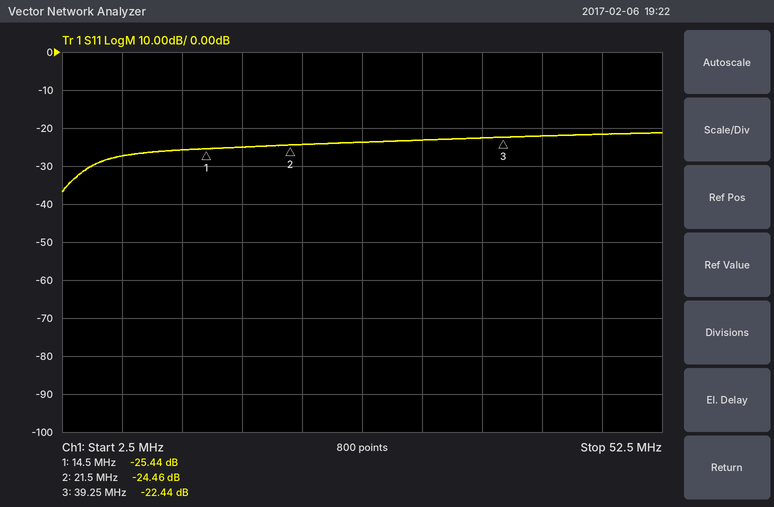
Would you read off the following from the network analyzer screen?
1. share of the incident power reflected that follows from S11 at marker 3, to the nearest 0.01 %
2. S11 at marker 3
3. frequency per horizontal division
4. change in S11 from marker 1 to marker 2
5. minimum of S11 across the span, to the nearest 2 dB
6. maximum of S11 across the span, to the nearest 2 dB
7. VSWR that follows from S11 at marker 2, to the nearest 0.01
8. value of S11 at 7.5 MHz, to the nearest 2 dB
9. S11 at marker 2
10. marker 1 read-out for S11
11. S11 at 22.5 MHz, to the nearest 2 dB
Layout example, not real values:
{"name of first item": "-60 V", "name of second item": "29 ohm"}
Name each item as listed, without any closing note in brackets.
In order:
{"share of the incident power reflected that follows from S11 at marker 3, to the nearest 0.01 %": "0.57 %", "S11 at marker 3": "-22.44 dB", "frequency per horizontal division": "5 MHz", "change in S11 from marker 1 to marker 2": "0.98 dB", "minimum of S11 across the span, to the nearest 2 dB": "-36 dB", "maximum of S11 across the span, to the nearest 2 dB": "-22 dB", "VSWR that follows from S11 at marker 2, to the nearest 0.01": "1.13", "value of S11 at 7.5 MHz, to the nearest 2 dB": "-28 dB", "S11 at marker 2": "-24.46 dB", "marker 1 read-out for S11": "-25.44 dB", "S11 at 22.5 MHz, to the nearest 2 dB": "-24 dB"}
